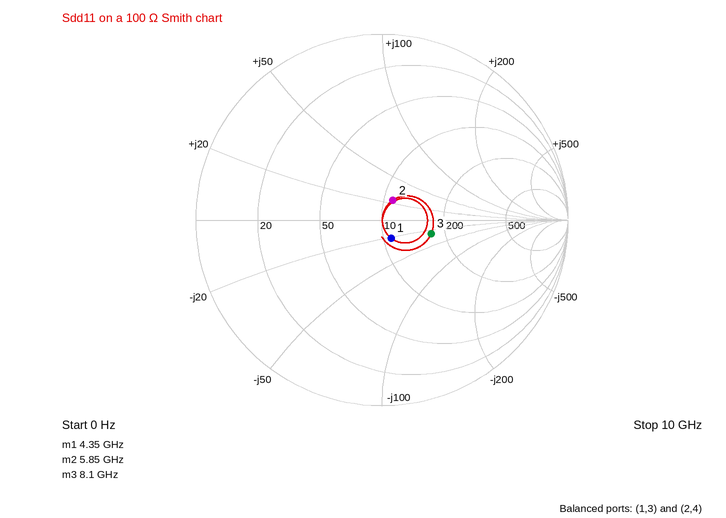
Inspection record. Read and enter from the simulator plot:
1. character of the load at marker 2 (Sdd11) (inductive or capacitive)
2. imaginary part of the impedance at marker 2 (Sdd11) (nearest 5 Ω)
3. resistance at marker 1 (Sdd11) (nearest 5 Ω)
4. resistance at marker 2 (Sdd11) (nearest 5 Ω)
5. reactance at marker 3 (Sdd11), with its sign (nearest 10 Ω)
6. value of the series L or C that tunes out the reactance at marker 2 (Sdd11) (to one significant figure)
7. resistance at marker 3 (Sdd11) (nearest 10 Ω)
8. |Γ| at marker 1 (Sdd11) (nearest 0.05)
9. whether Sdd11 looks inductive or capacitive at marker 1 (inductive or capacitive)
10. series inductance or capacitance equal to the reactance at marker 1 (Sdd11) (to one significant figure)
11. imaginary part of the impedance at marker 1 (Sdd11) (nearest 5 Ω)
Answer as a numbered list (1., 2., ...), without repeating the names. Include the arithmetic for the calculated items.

1. inductive
2. +25 Ω
3. 110 Ω
4. 110 Ω
5. -30 Ω
6. C = 1/(2π × 5.85 GHz × 25 Ω) ≈ 1 pF
7. 170 Ω
8. 0.10
9. capacitive
10. C = 1/(2π × 4.35 GHz × 20 Ω) ≈ 2 pF
11. -20 Ω
